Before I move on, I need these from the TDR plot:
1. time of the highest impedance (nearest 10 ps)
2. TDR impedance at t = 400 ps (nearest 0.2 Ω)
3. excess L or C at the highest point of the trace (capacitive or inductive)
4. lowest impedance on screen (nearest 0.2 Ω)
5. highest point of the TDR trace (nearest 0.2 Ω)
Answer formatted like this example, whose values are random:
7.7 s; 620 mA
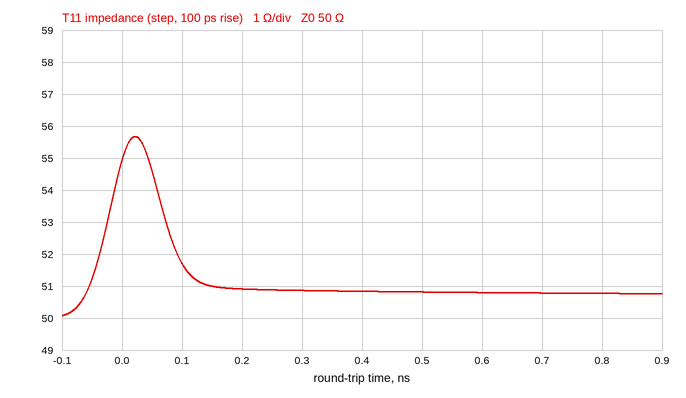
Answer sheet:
20 ps; 50.8 Ω; inductive; 50.0 Ω; 55.6 Ω
